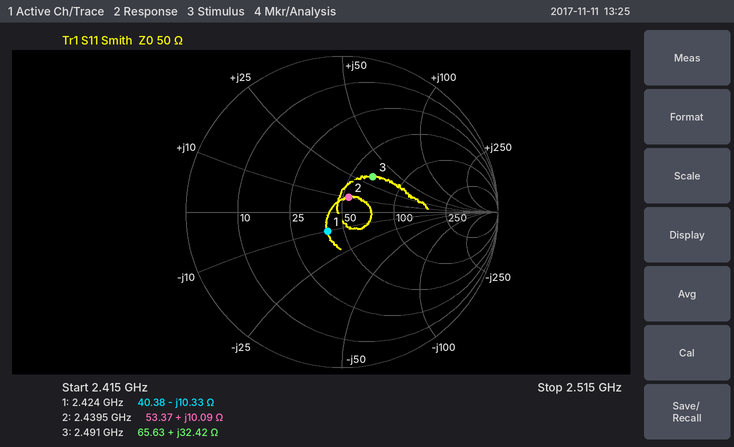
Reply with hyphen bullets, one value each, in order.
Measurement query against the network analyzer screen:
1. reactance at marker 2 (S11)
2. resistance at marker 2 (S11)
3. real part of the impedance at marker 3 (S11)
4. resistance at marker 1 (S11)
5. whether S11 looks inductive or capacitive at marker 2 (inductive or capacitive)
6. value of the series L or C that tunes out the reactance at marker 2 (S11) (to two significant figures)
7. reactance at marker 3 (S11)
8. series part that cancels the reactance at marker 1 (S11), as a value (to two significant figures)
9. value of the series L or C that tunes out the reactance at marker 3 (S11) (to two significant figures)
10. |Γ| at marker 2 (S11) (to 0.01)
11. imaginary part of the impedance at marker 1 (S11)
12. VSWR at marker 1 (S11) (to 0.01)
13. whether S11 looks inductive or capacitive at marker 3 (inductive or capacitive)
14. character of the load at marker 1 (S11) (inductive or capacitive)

- +10.09 Ω
- 53.37 Ω
- 65.63 Ω
- 40.38 Ω
- inductive
- 6.5 pF
- +32.42 Ω
- 680 pH
- 2.0 pF
- 0.10
- -10.33 Ω
- 1.37
- inductive
- capacitive
